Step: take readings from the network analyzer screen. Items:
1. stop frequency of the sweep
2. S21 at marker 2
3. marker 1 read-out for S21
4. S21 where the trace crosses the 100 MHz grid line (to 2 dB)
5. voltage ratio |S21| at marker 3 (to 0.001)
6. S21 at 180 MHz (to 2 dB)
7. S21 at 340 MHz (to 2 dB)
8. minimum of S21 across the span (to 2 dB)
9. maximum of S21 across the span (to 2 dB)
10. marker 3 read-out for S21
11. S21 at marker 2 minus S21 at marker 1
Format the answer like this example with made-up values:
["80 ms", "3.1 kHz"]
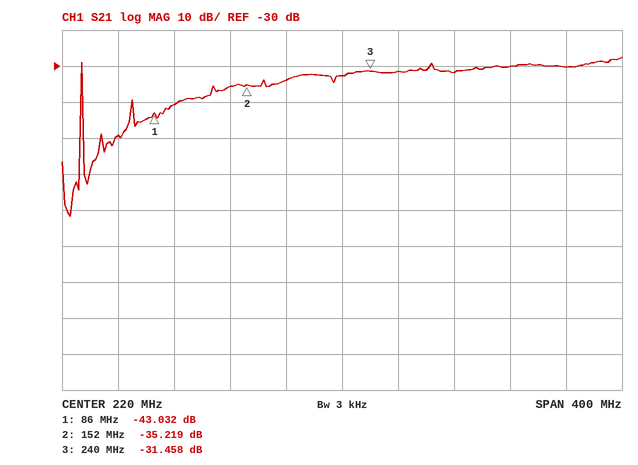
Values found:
["420 MHz", "-35.219 dB", "-43.032 dB", "-40 dB", "0.027", "-34 dB", "-30 dB", "-72 dB", "-28 dB", "-31.458 dB", "7.813 dB"]
